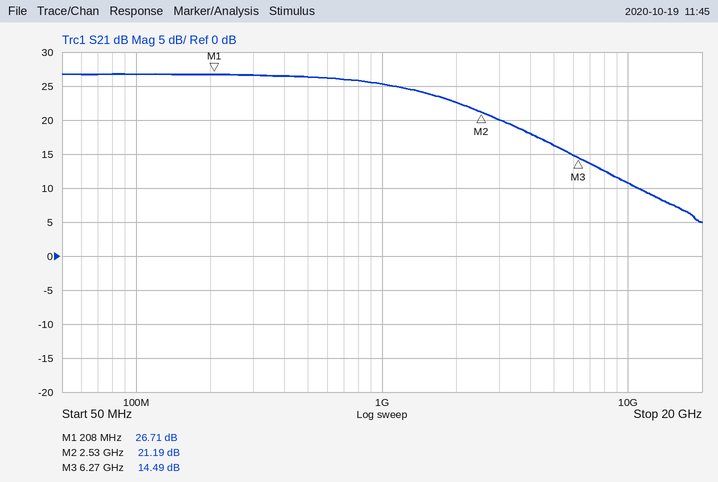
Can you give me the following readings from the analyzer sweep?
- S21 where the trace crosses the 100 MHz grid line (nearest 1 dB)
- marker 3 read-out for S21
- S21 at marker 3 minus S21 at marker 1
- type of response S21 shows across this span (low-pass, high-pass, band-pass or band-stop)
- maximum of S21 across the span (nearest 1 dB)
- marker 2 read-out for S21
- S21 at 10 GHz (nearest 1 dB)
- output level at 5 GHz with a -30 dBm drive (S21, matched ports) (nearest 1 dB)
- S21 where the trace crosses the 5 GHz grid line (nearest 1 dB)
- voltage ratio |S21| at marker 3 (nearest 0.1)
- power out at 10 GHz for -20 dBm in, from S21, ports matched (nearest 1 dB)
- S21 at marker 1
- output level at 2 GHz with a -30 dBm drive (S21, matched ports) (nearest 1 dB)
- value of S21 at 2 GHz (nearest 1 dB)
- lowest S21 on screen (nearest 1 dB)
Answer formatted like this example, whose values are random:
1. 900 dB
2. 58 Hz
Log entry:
1. 27 dB
2. 14.49 dB
3. -12.22 dB
4. low-pass
5. 27 dB
6. 21.19 dB
7. 11 dB
8. -14 dBm
9. 16 dB
10. 5.3
11. -9 dBm
12. 26.71 dB
13. -7 dBm
14. 23 dB
15. 5 dB
